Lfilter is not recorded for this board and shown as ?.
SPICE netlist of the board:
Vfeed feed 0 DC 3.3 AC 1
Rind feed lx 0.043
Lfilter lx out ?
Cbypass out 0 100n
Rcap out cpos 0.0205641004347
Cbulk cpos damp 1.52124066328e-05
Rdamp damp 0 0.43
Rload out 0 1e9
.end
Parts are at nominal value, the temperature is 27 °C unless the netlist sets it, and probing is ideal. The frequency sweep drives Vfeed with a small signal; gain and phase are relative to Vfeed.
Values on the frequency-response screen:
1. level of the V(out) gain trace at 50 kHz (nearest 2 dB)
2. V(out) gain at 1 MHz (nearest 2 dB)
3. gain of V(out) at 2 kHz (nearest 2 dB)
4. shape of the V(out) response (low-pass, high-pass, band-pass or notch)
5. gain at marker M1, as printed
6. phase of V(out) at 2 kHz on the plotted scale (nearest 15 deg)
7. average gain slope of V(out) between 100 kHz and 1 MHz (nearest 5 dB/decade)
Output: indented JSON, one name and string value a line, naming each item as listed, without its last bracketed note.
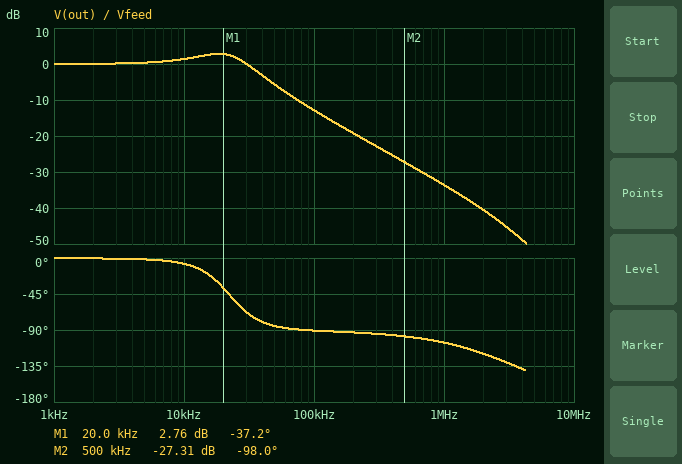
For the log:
{
  "level of the V(out) gain trace at 50 kHz": "-6 dB",
  "V(out) gain at 1 MHz": "-34 dB",
  "gain of V(out) at 2 kHz": "0 dB",
  "shape of the V(out) response": "low-pass",
  "gain at marker M1, as printed": "2.76 dB",
  "phase of V(out) at 2 kHz on the plotted scale": "0 deg",
  "average gain slope of V(out) between 100 kHz and 1 MHz": "-20 dB/decade"
}
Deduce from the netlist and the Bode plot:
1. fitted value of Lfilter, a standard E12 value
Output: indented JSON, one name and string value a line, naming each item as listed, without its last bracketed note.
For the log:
{
  "fitted value of Lfilter, a standard E12 value": "3.3 µH"
}
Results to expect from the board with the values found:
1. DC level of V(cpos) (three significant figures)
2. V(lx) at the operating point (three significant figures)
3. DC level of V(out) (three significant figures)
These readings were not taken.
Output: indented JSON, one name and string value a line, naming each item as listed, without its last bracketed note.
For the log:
{
  "DC level of V(cpos)": "3.30 V",
  "V(lx) at the operating point": "3.30 V",
  "DC level of V(out)": "3.30 V"
}
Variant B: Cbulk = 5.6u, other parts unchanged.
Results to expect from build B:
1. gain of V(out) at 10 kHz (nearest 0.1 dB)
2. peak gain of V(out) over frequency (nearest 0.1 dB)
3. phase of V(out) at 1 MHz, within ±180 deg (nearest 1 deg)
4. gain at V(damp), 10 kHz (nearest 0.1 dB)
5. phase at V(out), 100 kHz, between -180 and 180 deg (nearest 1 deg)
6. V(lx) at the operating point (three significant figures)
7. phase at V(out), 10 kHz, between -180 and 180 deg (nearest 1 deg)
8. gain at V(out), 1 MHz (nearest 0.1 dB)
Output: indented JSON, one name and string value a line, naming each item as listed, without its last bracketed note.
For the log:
{
  "gain of V(out) at 10 kHz": "0.6 dB",
  "peak gain of V(out) over frequency": "5.5 dB",
  "phase of V(out) at 1 MHz, within ±180 deg": "-108 deg",
  "gain at V(damp), 10 kHz": "-15.9 dB",
  "phase at V(out), 100 kHz, between -180 and 180 deg": "-109 deg",
  "V(lx) at the operating point": "3.30 V",
  "phase at V(out), 10 kHz, between -180 and 180 deg": "-2 deg",
  "gain at V(out), 1 MHz": "-33.7 dB"
}
